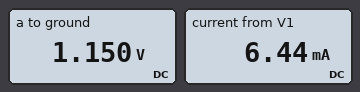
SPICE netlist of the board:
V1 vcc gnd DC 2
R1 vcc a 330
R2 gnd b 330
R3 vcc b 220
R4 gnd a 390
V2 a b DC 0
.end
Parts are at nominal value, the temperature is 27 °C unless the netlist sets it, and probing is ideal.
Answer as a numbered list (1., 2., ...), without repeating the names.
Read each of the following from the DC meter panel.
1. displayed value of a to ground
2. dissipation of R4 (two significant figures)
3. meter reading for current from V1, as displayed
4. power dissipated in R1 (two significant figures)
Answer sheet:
1. 1.150 V
2. 3.4 mW
3. 6.44 mA
4. 2.2 mW
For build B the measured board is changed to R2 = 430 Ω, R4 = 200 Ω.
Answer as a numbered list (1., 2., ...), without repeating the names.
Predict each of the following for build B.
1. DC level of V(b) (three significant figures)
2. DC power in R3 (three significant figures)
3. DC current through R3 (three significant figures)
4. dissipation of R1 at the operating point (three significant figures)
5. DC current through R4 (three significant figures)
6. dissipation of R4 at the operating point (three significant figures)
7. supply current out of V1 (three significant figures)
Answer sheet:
1. 1.02 V
2. 4.39 mW
3. 4.47 mA
4. 2.93 mW
5. 5.08 mA
6. 5.17 mW
7. 7.45 mA
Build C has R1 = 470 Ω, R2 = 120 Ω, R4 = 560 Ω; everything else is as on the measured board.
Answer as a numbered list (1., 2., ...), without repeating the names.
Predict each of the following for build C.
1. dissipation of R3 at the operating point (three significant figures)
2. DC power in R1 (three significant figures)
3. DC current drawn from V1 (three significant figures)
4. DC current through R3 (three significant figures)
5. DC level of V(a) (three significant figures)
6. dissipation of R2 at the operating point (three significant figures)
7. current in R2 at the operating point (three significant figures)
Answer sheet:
1. 6.60 mW
2. 3.09 mW
3. 8.04 mA
4. 5.48 mA
5. 795 mV
6. 5.26 mW
7. 6.62 mA
